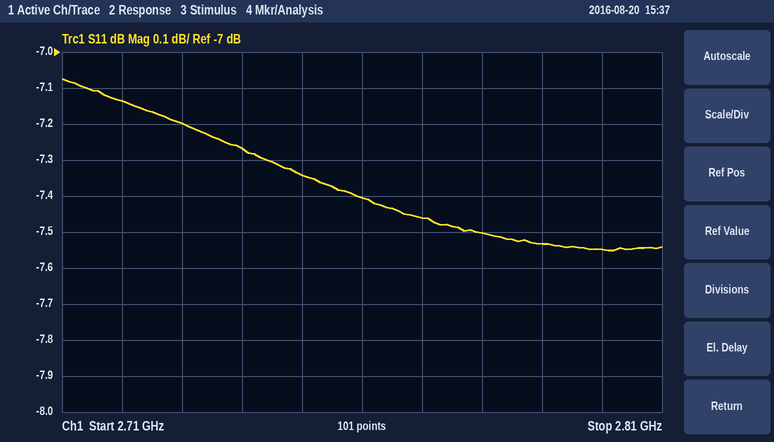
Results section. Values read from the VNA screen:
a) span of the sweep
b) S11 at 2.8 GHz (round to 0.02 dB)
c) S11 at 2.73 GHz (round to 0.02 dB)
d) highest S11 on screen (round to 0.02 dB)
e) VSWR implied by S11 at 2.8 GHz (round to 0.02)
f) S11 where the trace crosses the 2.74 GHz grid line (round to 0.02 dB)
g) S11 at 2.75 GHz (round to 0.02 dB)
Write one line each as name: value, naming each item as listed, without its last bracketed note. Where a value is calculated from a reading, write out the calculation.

span of the sweep: 100 MHz
S11 at 2.8 GHz: -7.54 dB
S11 at 2.73 GHz: -7.20 dB
highest S11 on screen: -7.08 dB
VSWR implied by S11 at 2.8 GHz: |Γ| = 10^(-7.54/20) = 0.4198; VSWR = (1 + 0.4198)/(1 − 0.4198) ≈ 2.45, so 2.44 to the nearest 0.02
S11 where the trace crosses the 2.74 GHz grid line: -7.26 dB
S11 at 2.75 GHz: -7.34 dB
